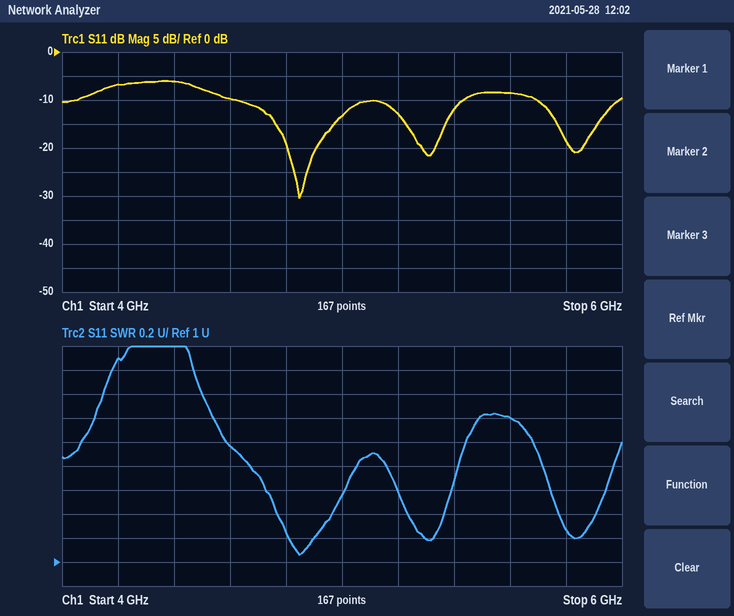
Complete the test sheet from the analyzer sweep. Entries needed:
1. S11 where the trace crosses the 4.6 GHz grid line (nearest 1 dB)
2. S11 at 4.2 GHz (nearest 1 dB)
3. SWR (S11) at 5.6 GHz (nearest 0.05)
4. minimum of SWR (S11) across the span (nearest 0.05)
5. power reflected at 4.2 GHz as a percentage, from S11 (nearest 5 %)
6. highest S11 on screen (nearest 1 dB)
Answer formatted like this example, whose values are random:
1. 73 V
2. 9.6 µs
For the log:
1. -10 dB
2. -7 dB
3. 2.20
4. 1.05
5. 20 %
6. -6 dB
